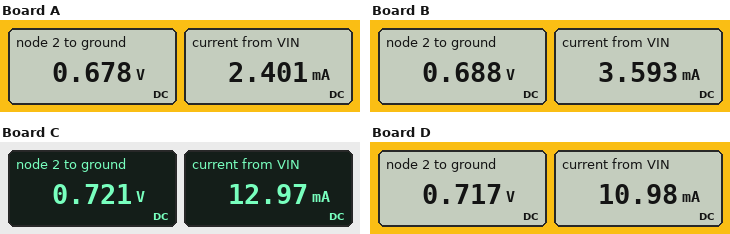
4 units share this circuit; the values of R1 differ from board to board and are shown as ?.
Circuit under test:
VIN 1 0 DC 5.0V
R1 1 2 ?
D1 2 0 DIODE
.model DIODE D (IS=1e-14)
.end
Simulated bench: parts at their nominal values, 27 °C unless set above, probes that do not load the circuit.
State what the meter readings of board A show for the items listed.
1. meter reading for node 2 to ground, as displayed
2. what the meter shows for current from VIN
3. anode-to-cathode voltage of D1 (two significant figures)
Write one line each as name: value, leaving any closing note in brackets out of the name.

meter reading for node 2 to ground, as displayed: 0.678 V
what the meter shows for current from VIN: 2.401 mA
anode-to-cathode voltage of D1: 680 mV
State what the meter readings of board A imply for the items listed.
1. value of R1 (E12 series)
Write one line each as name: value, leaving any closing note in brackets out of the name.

value of R1: 1.8 kΩ
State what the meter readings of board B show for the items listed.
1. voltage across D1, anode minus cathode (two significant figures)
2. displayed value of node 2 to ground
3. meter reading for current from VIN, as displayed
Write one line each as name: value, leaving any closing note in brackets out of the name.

voltage across D1, anode minus cathode: 690 mV
displayed value of node 2 to ground: 0.688 V
meter reading for current from VIN, as displayed: 3.593 mA
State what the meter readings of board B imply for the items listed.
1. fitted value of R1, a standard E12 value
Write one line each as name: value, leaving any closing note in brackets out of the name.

fitted value of R1, a standard E12 value: 1.2 kΩ
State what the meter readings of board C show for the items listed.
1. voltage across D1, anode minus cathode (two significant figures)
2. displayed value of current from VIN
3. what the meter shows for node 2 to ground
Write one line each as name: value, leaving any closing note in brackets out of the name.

voltage across D1, anode minus cathode: 720 mV
displayed value of current from VIN: 12.97 mA
what the meter shows for node 2 to ground: 0.721 V
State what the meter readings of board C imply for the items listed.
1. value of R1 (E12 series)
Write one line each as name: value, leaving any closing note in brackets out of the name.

value of R1: 330 Ω
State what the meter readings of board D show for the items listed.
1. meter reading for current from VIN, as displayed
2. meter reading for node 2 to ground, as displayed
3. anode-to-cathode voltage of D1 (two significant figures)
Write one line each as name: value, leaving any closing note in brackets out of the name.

meter reading for current from VIN, as displayed: 10.98 mA
meter reading for node 2 to ground, as displayed: 0.717 V
anode-to-cathode voltage of D1: 720 mV
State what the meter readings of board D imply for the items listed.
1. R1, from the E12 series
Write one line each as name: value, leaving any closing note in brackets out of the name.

R1, from the E12 series: 390 Ω
